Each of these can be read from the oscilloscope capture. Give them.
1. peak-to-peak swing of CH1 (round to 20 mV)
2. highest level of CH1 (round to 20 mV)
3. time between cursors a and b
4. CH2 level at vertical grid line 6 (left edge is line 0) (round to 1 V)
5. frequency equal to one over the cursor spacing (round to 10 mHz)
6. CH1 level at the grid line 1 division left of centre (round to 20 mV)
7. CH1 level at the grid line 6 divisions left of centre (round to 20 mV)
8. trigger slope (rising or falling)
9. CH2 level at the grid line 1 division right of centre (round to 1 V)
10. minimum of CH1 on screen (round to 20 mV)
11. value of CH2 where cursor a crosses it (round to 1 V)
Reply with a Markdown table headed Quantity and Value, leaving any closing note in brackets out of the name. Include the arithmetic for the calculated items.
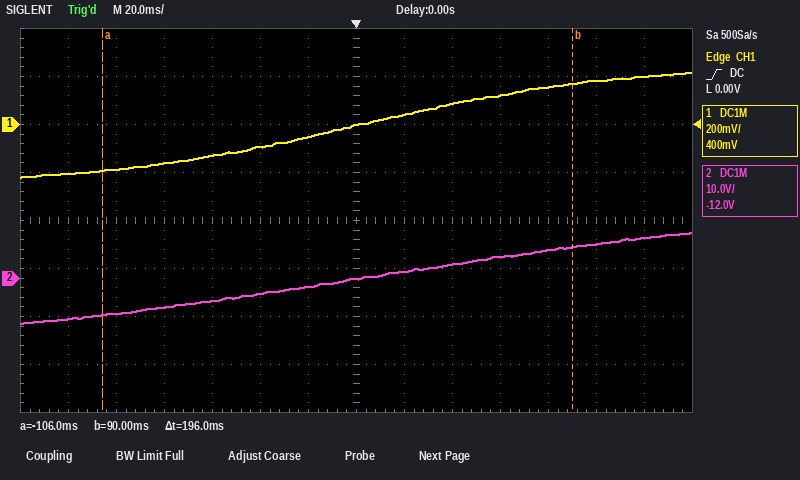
| Quantity | Value |
|---|---|
| peak-to-peak swing of CH1 | 220 mV − (-220 mV) = 440 mV |
| highest level of CH1 | 220 mV |
| time between cursors a and b | 196 ms |
| CH2 level at vertical grid line 6 (left edge is line 0) | -2 V |
| frequency equal to one over the cursor spacing | 1 / 196 ms ≈ 5.10 Hz |
| CH1 level at the grid line 1 division left of centre | -60 mV |
| CH1 level at the grid line 6 divisions left of centre | -200 mV |
| trigger slope | rising |
| CH2 level at the grid line 1 division right of centre | 1 V |
| minimum of CH1 on screen | -220 mV |
| value of CH2 where cursor a crosses it | -8 V |
